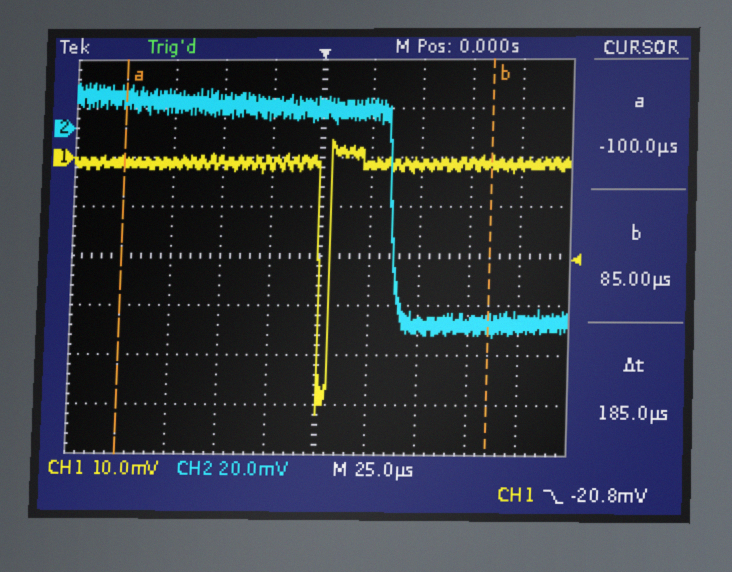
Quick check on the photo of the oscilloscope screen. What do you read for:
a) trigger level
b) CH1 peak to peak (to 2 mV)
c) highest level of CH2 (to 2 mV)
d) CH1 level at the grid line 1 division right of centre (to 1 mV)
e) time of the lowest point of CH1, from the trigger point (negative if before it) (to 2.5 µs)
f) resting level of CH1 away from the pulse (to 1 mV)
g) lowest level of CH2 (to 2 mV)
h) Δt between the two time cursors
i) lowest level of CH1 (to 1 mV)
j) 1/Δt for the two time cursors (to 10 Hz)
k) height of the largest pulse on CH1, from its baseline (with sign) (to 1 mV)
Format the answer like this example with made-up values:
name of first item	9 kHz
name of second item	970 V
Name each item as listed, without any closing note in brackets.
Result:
trigger level	-20.8 mV
CH1 peak to peak	56 mV
highest level of CH2	18 mV
CH1 level at the grid line 1 division right of centre	-2 mV
time of the lowest point of CH1, from the trigger point (negative if before it)	0.0 µs
resting level of CH1 away from the pulse	-1 mV
lowest level of CH2	-84 mV
Δt between the two time cursors	185 µs
lowest level of CH1	-52 mV
1/Δt for the two time cursors	5.41 kHz
height of the largest pulse on CH1, from its baseline (with sign)	-51 mV
